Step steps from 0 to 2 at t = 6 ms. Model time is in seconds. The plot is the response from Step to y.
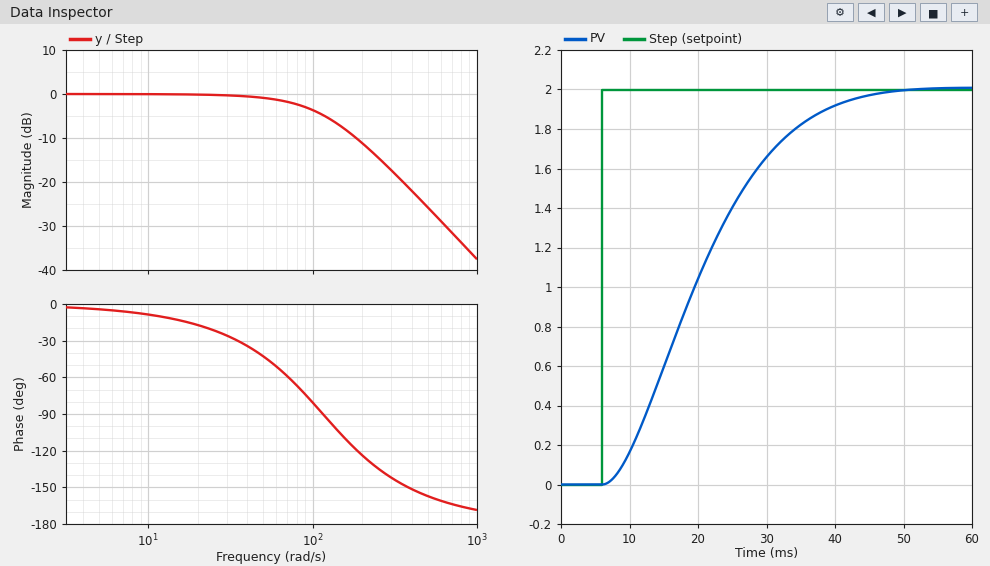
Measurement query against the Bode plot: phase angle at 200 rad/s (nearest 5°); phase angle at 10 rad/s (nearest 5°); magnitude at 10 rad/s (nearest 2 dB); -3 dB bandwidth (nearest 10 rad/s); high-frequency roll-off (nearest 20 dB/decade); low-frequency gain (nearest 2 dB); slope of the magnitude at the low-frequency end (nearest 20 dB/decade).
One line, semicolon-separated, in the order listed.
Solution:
-125°; -10°; 0 dB; 90 rad/s; -40 dB/decade; 0 dB; 0 dB/decade
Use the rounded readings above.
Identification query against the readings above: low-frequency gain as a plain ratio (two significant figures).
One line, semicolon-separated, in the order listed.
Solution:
1.0
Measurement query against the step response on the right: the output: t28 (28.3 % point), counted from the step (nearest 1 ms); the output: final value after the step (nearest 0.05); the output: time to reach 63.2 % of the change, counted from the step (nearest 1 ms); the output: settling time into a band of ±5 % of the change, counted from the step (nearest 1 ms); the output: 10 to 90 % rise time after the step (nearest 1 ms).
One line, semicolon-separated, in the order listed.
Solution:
9 ms; 2.00; 17 ms; 33 ms; 24 ms
